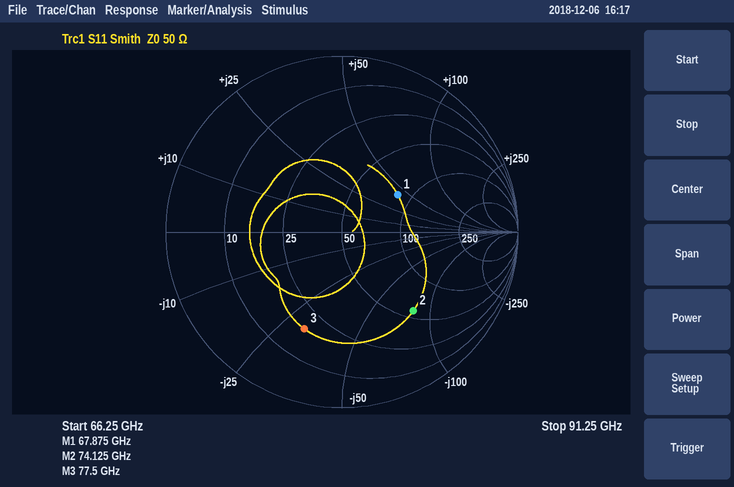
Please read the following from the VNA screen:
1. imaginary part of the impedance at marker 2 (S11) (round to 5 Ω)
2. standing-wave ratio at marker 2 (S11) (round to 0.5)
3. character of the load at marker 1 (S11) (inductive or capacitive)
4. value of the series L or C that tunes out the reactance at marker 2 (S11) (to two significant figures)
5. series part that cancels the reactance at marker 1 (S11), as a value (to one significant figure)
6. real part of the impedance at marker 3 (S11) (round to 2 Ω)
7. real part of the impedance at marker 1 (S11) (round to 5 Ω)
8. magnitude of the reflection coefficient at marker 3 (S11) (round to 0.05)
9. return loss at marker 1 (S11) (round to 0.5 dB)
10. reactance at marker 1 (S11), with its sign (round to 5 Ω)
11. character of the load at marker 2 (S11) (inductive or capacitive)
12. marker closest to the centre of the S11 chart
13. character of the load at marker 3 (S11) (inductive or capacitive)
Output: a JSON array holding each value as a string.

["-80 Ω", "4.0", "inductive", "170 pH", "60 fF", "18 Ω", "85 Ω", "0.60", "8.5 dB", "+40 Ω", "capacitive", "marker 1", "capacitive"]
